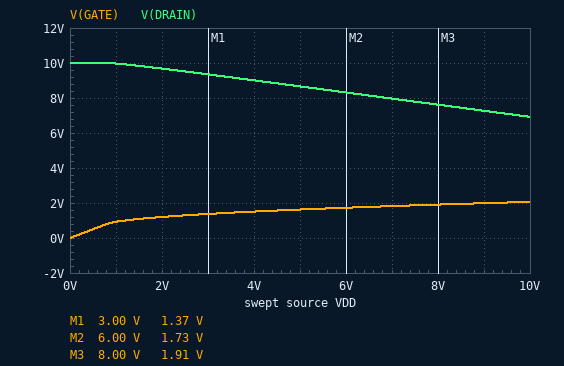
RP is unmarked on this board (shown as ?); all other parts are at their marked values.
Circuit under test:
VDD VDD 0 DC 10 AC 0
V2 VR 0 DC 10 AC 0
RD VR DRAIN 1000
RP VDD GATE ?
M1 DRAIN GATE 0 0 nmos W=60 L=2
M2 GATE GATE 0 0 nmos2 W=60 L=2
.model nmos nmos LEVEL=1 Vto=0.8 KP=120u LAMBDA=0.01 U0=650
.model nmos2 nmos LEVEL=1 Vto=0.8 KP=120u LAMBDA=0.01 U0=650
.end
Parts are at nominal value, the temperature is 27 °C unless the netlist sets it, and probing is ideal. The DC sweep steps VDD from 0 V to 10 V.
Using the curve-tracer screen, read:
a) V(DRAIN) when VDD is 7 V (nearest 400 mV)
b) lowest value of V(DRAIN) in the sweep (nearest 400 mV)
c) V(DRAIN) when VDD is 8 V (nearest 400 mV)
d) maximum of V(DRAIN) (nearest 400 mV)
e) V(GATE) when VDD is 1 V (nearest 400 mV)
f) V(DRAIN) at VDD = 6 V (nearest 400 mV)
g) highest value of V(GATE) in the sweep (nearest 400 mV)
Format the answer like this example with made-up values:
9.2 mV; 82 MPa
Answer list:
8.0 V; 6.8 V; 7.6 V; 10.0 V; 800 mV; 8.4 V; 2.0 V
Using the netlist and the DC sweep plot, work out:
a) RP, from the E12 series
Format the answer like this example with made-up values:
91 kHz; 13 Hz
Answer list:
2.7 kΩ
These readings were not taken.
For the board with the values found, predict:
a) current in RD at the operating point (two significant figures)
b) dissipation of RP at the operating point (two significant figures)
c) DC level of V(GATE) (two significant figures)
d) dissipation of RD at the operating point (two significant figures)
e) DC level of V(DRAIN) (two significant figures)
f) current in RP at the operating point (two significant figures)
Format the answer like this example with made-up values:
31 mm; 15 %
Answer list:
3.1 mA; 23 mW; 2.1 V; 9.5 mW; 6.9 V; 2.9 mA
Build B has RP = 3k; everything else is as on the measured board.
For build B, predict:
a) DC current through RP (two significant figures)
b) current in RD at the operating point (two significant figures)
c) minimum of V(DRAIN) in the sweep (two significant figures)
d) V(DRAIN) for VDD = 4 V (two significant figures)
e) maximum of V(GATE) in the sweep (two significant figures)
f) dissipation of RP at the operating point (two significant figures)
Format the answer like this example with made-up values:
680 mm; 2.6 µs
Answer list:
2.7 mA; 2.8 mA; 7.2 V; 9.1 V; 2.0 V; 21 mW
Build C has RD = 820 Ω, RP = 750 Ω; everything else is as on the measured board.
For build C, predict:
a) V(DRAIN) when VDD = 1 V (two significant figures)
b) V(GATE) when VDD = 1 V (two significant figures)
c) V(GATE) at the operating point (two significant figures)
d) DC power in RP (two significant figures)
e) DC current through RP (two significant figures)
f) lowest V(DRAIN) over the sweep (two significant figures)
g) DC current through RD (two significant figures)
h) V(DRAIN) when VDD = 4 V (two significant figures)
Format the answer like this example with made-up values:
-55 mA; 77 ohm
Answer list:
10 V; 960 mV; 3.0 V; 65 mW; 9.3 mA; 2.4 V; 9.2 mA; 7.7 V
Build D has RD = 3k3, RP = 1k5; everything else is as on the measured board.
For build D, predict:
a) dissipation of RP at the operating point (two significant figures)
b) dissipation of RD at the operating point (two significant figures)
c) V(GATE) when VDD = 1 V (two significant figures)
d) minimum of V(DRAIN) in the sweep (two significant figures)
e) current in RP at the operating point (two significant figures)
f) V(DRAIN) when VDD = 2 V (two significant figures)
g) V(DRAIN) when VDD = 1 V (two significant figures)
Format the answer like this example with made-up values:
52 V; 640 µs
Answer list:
38 mW; 27 mW; 940 mV; 580 mV; 5.0 mA; 8.4 V; 9.9 V
